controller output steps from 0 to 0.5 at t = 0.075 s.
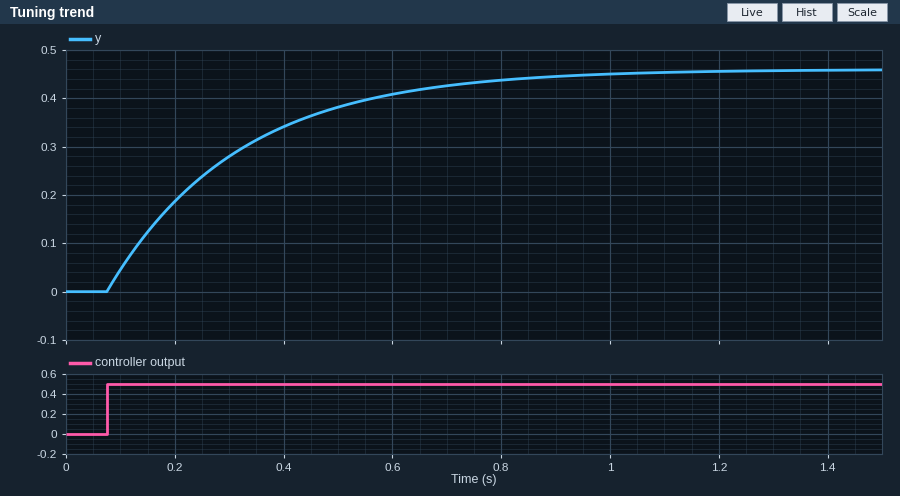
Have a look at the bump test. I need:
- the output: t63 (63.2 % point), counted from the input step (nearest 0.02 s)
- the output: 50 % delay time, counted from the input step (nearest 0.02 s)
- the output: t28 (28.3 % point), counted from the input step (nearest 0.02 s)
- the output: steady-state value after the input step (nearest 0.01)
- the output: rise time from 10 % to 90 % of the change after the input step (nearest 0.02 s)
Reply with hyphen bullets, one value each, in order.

- 0.24 s
- 0.16 s
- 0.08 s
- 0.46
- 0.52 s
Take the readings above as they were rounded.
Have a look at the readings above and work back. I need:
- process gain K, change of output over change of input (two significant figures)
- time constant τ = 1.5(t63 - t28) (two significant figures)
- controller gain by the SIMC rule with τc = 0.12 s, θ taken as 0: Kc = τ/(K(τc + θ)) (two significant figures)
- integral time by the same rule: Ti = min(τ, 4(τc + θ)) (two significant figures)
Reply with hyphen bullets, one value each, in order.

- 0.92
- 0.24 s
- 2.2
- 0.24 s
